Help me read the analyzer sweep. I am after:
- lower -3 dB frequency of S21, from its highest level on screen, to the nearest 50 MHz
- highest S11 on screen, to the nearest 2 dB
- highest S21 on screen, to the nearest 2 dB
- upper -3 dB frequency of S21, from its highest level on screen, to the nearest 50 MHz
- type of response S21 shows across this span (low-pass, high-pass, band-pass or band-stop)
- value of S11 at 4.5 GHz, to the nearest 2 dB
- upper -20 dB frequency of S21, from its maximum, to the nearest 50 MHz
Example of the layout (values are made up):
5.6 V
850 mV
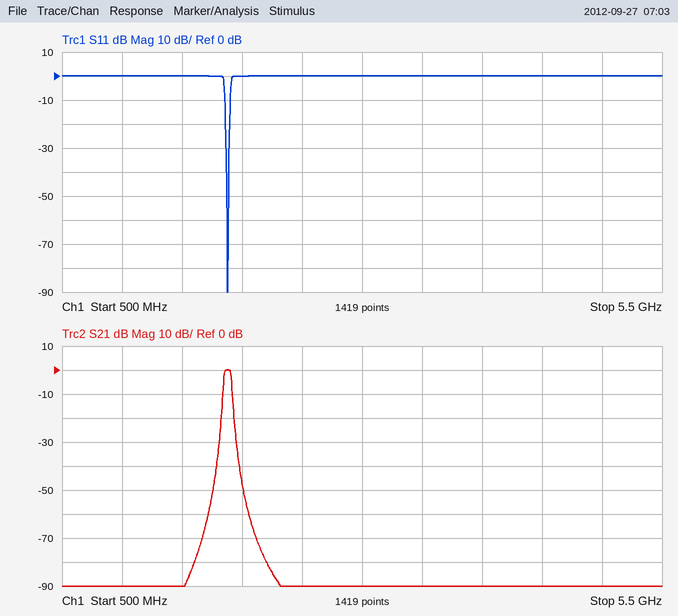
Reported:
1.85 GHz
0 dB
0 dB
1.90 GHz
band-pass
0 dB
1.95 GHz
